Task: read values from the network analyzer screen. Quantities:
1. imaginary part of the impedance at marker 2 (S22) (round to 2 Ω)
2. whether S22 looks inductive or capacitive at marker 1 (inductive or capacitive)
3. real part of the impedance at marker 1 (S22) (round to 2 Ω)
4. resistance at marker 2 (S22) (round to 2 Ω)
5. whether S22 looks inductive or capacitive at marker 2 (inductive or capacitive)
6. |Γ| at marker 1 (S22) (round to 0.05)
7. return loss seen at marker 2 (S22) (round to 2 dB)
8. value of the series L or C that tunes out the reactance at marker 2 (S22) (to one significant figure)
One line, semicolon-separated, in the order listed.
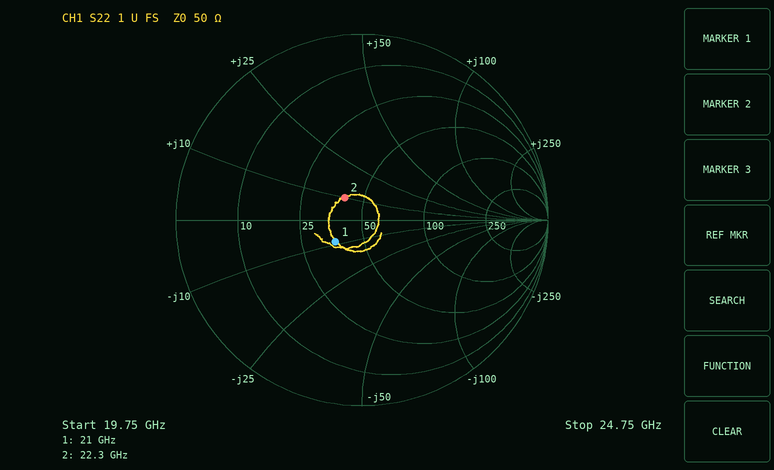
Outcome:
+10 Ω; capacitive; 36 Ω; 40 Ω; inductive; 0.20; 16 dB; 700 fF
